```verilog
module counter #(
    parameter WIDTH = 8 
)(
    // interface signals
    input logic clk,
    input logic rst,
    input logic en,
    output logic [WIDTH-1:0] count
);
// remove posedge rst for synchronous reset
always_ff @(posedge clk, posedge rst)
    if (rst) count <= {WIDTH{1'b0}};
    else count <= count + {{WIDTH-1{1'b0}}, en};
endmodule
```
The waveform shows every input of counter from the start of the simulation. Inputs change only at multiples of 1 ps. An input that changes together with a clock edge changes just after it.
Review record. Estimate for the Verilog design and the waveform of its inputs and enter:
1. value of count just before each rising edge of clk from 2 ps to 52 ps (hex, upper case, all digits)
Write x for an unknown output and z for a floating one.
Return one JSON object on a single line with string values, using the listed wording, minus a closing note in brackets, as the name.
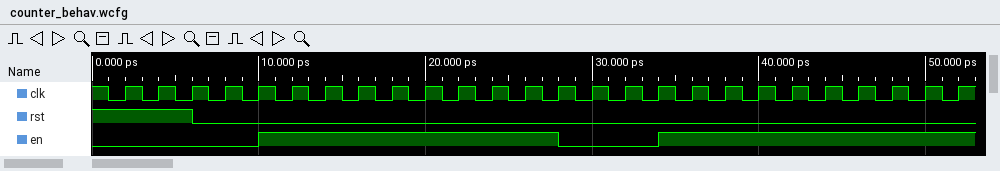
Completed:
{"value of count just before each rising edge of clk from 2 ps to 52 ps": "00, 00, 00, 00, 00, 00, 01, 02, 03, 04, 05, 06, 07, 08, 09, 09, 09, 09, 0A, 0B, 0C, 0D, 0E, 0F, 10, 11"}
